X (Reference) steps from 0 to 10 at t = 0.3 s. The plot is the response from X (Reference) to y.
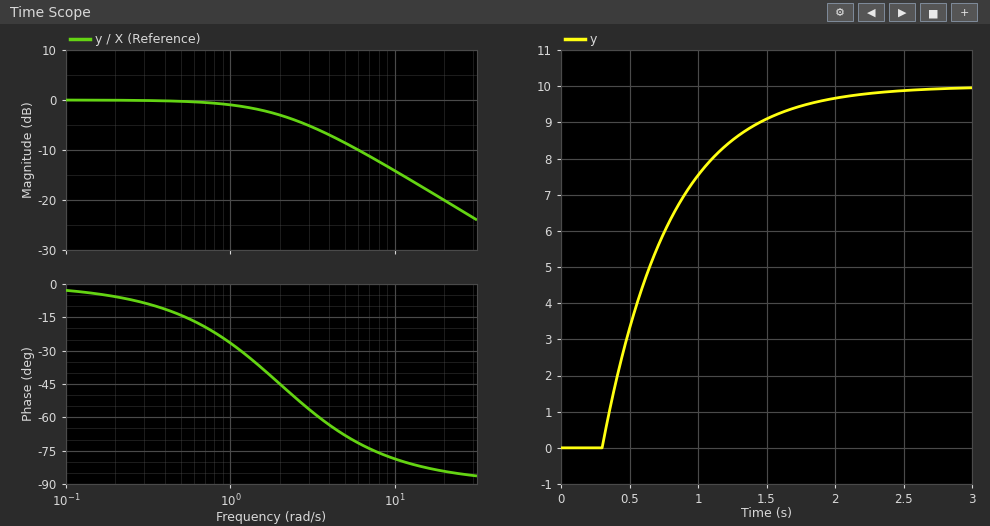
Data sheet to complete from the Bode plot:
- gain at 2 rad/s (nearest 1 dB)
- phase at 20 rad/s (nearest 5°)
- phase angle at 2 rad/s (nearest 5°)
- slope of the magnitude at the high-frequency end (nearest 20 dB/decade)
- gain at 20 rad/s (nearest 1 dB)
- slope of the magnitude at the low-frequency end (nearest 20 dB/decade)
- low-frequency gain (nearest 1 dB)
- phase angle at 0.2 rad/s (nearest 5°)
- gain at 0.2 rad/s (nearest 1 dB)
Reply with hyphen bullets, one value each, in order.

- -3 dB
- -85°
- -45°
- -20 dB/decade
- -20 dB
- 0 dB/decade
- 0 dB
- -5°
- 0 dB
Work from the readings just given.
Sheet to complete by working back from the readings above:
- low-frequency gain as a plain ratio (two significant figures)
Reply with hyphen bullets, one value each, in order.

- 1.0
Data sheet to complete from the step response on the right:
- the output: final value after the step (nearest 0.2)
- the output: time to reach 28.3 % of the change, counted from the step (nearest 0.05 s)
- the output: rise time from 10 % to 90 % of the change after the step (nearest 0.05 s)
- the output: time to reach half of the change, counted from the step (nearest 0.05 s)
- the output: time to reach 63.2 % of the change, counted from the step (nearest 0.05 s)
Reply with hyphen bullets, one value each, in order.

- 10.0
- 0.15 s
- 1.10 s
- 0.35 s
- 0.50 s
